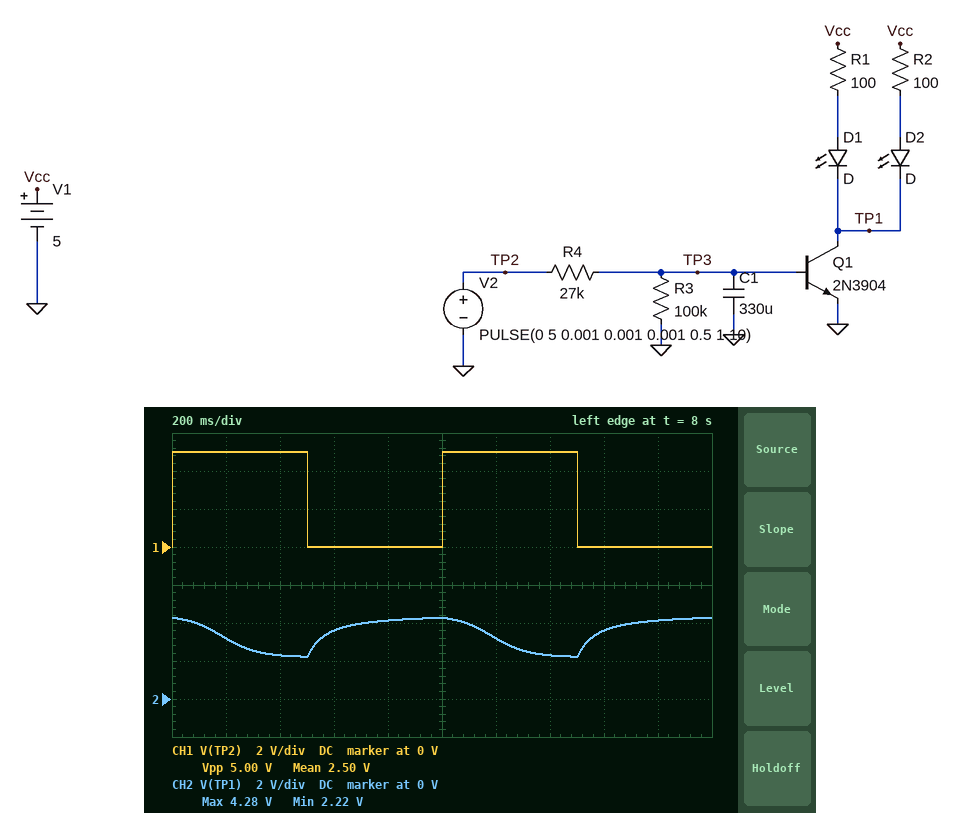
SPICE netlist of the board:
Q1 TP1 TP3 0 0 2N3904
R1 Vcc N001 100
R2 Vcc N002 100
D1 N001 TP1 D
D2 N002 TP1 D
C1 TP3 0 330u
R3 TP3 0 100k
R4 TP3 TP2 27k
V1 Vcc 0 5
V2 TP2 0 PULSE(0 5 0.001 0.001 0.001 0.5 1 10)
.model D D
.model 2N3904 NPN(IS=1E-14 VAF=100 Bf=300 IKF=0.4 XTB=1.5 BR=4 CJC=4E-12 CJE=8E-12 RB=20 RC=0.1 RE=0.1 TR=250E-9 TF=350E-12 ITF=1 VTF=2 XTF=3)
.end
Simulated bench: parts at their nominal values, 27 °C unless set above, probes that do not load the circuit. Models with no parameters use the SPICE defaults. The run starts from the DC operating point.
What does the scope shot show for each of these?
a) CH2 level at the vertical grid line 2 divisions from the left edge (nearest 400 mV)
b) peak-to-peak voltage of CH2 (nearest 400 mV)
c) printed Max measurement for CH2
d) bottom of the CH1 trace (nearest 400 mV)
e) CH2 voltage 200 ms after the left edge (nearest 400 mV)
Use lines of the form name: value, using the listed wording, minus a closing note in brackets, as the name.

CH2 level at the vertical grid line 2 divisions from the left edge: 2.4 V
peak-to-peak voltage of CH2: 2.0 V
printed Max measurement for CH2: 4.28 V
bottom of the CH1 trace: 0 V
CH2 voltage 200 ms after the left edge: 3.2 V
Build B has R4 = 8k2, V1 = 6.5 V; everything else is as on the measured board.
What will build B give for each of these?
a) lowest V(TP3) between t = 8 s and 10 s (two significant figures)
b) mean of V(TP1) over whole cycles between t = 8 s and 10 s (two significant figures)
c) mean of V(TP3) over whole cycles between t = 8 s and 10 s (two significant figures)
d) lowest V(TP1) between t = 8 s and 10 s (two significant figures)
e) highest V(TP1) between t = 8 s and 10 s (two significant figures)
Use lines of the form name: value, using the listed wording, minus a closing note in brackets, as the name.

lowest V(TP3) between t = 8 s and 10 s: 610 mV
mean of V(TP1) over whole cycles between t = 8 s and 10 s: 3.4 V
mean of V(TP3) over whole cycles between t = 8 s and 10 s: 730 mV
lowest V(TP1) between t = 8 s and 10 s: 210 mV
highest V(TP1) between t = 8 s and 10 s: 5.9 V
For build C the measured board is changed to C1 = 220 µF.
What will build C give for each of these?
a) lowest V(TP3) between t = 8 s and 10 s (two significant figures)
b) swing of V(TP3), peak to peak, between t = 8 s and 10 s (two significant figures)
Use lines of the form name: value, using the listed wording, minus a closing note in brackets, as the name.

lowest V(TP3) between t = 8 s and 10 s: 640 mV
swing of V(TP3), peak to peak, between t = 8 s and 10 s: 120 mV
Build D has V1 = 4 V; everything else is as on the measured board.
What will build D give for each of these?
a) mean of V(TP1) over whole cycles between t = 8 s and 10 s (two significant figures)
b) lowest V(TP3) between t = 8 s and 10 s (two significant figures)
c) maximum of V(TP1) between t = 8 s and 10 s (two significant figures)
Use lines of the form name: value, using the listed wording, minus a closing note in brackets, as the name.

mean of V(TP1) over whole cycles between t = 8 s and 10 s: 2.5 V
lowest V(TP3) between t = 8 s and 10 s: 670 mV
maximum of V(TP1) between t = 8 s and 10 s: 3.3 V
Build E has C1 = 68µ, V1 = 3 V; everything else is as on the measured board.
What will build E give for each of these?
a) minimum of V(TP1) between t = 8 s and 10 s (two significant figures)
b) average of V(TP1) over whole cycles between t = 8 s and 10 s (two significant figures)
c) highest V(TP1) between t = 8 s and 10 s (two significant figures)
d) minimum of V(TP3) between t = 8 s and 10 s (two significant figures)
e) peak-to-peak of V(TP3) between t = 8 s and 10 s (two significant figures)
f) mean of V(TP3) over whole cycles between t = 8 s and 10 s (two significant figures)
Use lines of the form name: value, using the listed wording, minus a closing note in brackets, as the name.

minimum of V(TP1) between t = 8 s and 10 s: 250 mV
average of V(TP1) over whole cycles between t = 8 s and 10 s: 1.5 V
highest V(TP1) between t = 8 s and 10 s: 2.5 V
minimum of V(TP3) between t = 8 s and 10 s: 500 mV
peak-to-peak of V(TP3) between t = 8 s and 10 s: 260 mV
mean of V(TP3) over whole cycles between t = 8 s and 10 s: 670 mV
